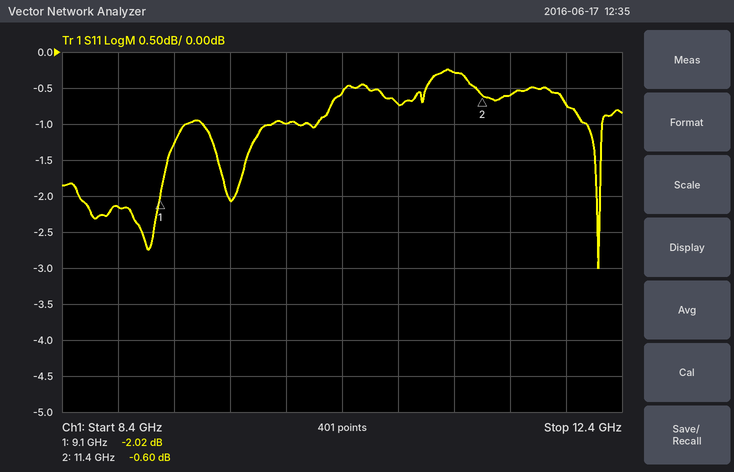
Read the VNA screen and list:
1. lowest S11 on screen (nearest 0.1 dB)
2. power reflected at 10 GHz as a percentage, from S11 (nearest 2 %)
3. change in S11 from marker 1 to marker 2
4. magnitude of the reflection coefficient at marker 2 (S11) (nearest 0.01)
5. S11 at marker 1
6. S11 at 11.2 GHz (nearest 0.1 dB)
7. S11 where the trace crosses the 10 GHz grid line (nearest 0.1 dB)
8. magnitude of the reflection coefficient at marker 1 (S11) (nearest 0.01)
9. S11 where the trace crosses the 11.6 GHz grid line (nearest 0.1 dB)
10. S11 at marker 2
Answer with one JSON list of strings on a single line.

["-3.0 dB", "80 %", "1.42 dB", "0.93", "-2.02 dB", "-0.3 dB", "-1.0 dB", "0.79", "-0.6 dB", "-0.60 dB"]
